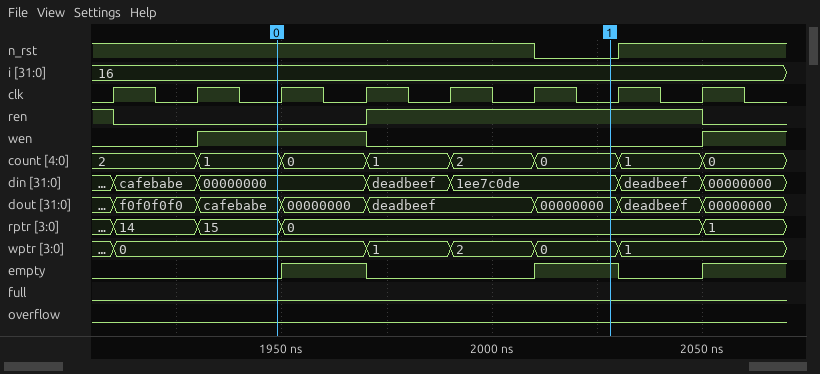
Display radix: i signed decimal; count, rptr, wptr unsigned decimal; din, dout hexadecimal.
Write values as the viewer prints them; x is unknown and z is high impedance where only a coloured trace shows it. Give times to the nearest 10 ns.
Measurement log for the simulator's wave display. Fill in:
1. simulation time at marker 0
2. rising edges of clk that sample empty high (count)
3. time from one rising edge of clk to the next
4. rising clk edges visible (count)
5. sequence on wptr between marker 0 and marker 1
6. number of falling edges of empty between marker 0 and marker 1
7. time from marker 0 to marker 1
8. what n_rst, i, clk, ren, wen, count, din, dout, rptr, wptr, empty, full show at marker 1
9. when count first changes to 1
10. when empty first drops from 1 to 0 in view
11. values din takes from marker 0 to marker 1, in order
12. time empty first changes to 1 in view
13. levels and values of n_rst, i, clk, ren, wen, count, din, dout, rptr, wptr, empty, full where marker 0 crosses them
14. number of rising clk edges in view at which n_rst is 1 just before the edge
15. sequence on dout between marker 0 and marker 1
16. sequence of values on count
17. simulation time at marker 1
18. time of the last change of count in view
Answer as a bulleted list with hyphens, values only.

- 1950 ns
- 2
- 20 ns
- 8
- 0, 1, 2, 0
- 1
- 80 ns
- n_rst=0, i=16, clk=0, ren=1, wen=0, count=0, din=1ee7c0de, dout=00000000, rptr=0, wptr=0, empty=1, full=0
- 1930 ns
- 1970 ns
- 00000000, deadbeef, 1ee7c0de
- 1950 ns
- n_rst=1, i=16, clk=0, ren=0, wen=1, count=1, din=00000000, dout=cafebabe, rptr=15, wptr=0, empty=0, full=0
- 7
- cafebabe, 00000000, deadbeef, 00000000
- 2, 1, 0, 1, 2, 0, 1, 0
- 2030 ns
- 2050 ns
